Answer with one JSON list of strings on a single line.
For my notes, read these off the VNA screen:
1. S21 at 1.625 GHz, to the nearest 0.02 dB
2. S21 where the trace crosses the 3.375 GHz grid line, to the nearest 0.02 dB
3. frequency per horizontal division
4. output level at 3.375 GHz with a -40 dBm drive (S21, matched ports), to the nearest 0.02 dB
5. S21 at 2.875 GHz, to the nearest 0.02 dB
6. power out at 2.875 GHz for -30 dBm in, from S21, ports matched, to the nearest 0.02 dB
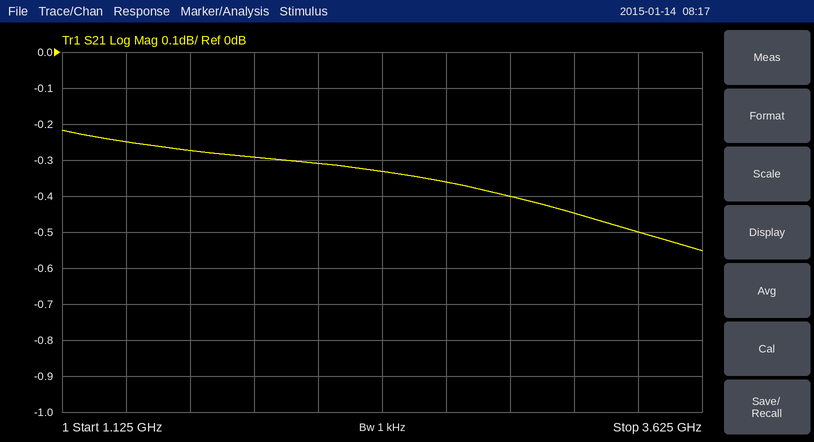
["-0.28 dB", "-0.50 dB", "250 MHz", "-40.50 dBm", "-0.40 dB", "-30.40 dBm"]
